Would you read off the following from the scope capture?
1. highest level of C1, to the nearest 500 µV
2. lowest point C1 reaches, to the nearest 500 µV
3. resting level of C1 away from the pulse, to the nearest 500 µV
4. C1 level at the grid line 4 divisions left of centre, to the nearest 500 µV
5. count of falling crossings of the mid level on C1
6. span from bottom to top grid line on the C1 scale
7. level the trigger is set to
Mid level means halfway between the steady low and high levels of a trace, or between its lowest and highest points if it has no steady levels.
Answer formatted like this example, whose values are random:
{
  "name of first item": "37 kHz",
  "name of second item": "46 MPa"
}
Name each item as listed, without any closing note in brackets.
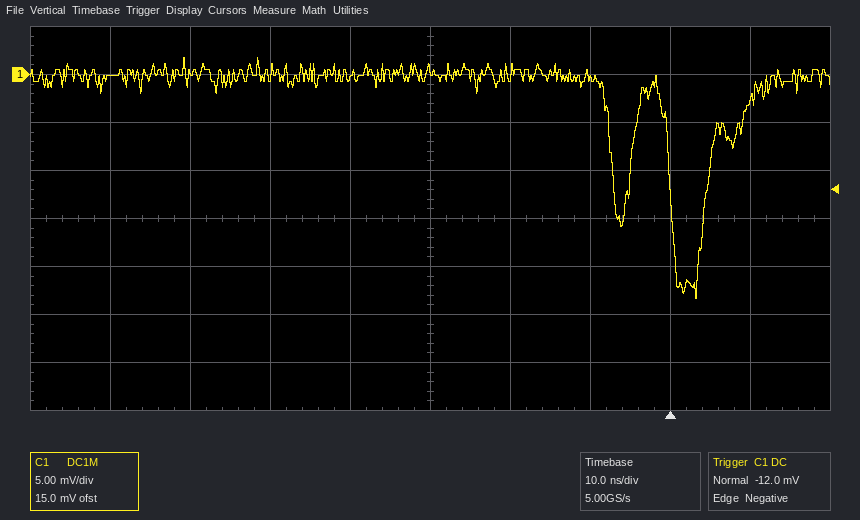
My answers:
{
  "highest level of C1, to the nearest 500 µV": "2.0 mV",
  "lowest point C1 reaches, to the nearest 500 µV": "-23.5 mV",
  "resting level of C1 away from the pulse, to the nearest 500 µV": "0.0 mV",
  "C1 level at the grid line 4 divisions left of centre, to the nearest 500 µV": "-500 µV",
  "count of falling crossings of the mid level on C1": "2",
  "span from bottom to top grid line on the C1 scale": "40 mV",
  "level the trigger is set to": "-12.0 mV"
}
